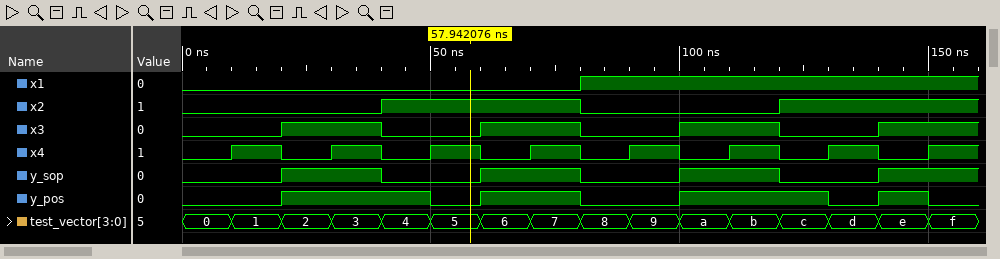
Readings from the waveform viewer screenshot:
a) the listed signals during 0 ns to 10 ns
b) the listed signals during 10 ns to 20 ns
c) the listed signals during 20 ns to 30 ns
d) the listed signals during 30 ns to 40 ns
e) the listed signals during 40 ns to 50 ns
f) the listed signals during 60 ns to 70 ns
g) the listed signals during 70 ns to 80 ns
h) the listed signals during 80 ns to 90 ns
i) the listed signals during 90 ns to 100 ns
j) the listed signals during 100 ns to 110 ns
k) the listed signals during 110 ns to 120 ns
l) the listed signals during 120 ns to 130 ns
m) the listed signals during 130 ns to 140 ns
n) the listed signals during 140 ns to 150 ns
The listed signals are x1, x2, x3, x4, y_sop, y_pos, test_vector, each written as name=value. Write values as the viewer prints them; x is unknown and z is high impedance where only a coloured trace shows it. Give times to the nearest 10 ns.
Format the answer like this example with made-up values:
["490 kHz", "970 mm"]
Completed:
["x1=0, x2=0, x3=0, x4=0, y_sop=0, y_pos=0, test_vector=0", "x1=0, x2=0, x3=0, x4=1, y_sop=0, y_pos=0, test_vector=1", "x1=0, x2=0, x3=1, x4=0, y_sop=1, y_pos=1, test_vector=2", "x1=0, x2=0, x3=1, x4=1, y_sop=1, y_pos=1, test_vector=3", "x1=0, x2=1, x3=0, x4=0, y_sop=0, y_pos=1, test_vector=4", "x1=0, x2=1, x3=1, x4=0, y_sop=1, y_pos=1, test_vector=6", "x1=0, x2=1, x3=1, x4=1, y_sop=1, y_pos=1, test_vector=7", "x1=1, x2=0, x3=0, x4=0, y_sop=0, y_pos=0, test_vector=8", "x1=1, x2=0, x3=0, x4=1, y_sop=0, y_pos=0, test_vector=9", "x1=1, x2=0, x3=1, x4=0, y_sop=1, y_pos=1, test_vector=a", "x1=1, x2=0, x3=1, x4=1, y_sop=1, y_pos=1, test_vector=b", "x1=1, x2=1, x3=0, x4=0, y_sop=0, y_pos=1, test_vector=c", "x1=1, x2=1, x3=0, x4=1, y_sop=0, y_pos=0, test_vector=d", "x1=1, x2=1, x3=1, x4=0, y_sop=1, y_pos=1, test_vector=e"]
